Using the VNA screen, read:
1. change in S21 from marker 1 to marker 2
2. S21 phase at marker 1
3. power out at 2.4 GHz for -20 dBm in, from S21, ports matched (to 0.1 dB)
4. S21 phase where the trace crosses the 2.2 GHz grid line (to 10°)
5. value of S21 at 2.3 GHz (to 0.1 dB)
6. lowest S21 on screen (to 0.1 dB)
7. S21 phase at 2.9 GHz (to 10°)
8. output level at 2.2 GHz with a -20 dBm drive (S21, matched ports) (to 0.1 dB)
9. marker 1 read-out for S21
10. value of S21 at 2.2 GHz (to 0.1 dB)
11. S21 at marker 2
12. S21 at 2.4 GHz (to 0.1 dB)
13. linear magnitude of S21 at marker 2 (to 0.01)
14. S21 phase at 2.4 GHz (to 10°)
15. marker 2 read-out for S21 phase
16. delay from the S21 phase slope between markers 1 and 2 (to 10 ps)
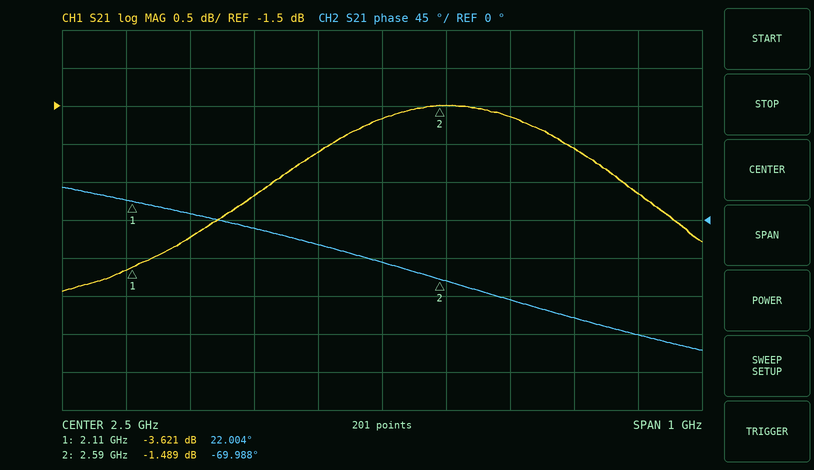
2.132 dB
22.004°
-22.1 dBm
10°
-2.7 dB
-3.9 dB
-140°
-23.2 dBm
-3.621 dB
-3.2 dB
-1.489 dB
-2.1 dB
0.84
-30°
-69.988°
530 ps
